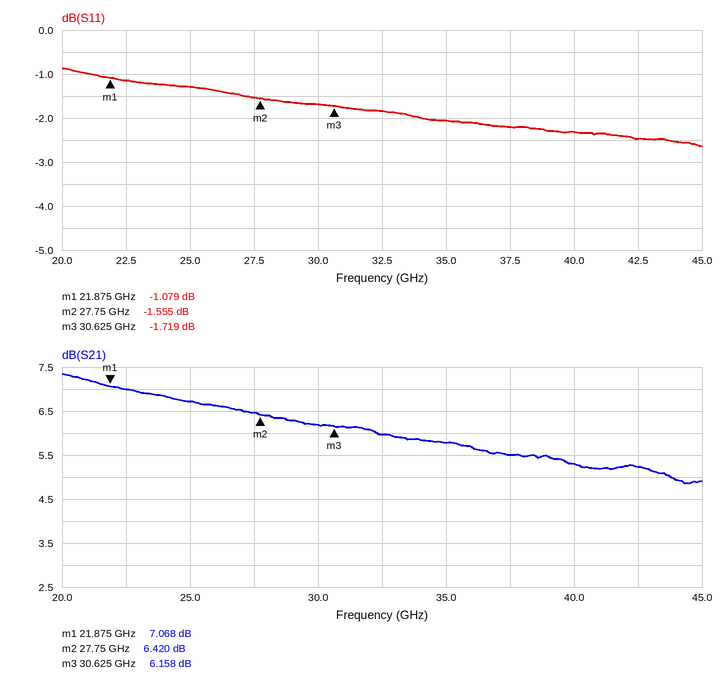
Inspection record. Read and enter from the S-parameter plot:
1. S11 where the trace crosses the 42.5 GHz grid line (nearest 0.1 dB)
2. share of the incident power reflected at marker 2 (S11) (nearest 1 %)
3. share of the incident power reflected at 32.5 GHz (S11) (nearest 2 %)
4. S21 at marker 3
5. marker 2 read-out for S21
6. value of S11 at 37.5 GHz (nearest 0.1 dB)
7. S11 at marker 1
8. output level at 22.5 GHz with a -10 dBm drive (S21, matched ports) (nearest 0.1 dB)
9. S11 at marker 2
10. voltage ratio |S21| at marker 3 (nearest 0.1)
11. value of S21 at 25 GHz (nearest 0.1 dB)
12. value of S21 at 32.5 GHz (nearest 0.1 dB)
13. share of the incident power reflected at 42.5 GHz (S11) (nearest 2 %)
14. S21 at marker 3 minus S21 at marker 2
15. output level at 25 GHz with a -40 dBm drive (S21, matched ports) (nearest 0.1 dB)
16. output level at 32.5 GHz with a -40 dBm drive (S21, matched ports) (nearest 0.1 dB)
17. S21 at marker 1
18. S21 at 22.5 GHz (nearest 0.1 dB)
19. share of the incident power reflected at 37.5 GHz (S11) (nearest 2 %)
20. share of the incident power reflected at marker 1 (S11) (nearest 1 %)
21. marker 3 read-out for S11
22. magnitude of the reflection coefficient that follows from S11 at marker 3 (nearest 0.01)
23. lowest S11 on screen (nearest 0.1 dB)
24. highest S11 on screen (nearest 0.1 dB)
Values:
-2.5 dB
70 %
66 %
6.158 dB
6.420 dB
-2.2 dB
-1.079 dB
-3.0 dBm
-1.555 dB
2.0
6.7 dB
6.0 dB
56 %
-0.262 dB
-33.3 dBm
-34.0 dBm
7.068 dB
7.0 dB
60 %
78 %
-1.719 dB
0.82
-2.6 dB
-0.9 dB
